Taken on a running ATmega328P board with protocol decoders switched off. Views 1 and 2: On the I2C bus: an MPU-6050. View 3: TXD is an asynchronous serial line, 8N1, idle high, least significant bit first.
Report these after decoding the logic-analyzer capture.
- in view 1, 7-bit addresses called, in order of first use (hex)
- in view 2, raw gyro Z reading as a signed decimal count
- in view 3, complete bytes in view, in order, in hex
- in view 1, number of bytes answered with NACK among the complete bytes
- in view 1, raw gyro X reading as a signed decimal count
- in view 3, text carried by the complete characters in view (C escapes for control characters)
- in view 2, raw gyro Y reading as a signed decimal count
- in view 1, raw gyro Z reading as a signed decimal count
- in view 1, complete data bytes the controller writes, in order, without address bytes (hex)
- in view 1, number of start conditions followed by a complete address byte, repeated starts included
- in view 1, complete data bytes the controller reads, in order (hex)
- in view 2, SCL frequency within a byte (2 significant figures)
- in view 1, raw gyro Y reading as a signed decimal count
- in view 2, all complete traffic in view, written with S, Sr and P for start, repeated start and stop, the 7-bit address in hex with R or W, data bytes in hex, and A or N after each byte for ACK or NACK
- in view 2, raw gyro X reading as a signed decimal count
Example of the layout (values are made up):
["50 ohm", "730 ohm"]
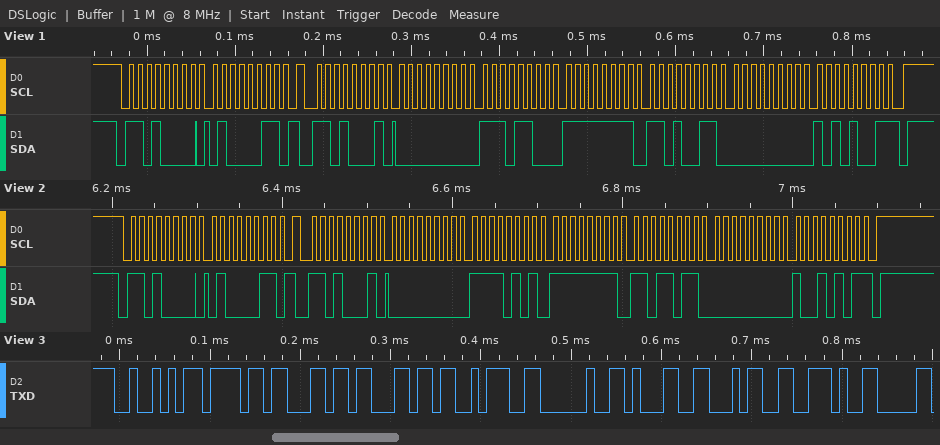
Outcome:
["0x68", "149", "52 6F 6C 6C 3A 20 31 34 2E", "1", "236", "\"Roll: 14.\"", "-37", "169", "43", "2", "00 EC FF D3 00 A9", "100 kHz", "-45", "S 68W A 43 A Sr 68R A 00 A F5 A FF A DB A 00 A 95 N P", "245"]
